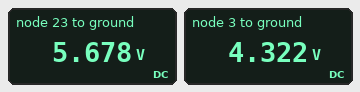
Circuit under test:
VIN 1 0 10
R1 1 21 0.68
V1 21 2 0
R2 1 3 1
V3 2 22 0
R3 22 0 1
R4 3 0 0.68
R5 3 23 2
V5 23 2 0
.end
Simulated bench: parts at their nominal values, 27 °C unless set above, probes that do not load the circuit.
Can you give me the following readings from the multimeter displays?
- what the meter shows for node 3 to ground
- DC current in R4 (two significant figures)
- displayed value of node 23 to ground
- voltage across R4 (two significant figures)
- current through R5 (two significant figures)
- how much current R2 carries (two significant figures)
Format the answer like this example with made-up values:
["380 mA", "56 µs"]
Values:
["4.322 V", "6.4 A", "5.678 V", "4.3 V", "680 mA", "5.7 A"]
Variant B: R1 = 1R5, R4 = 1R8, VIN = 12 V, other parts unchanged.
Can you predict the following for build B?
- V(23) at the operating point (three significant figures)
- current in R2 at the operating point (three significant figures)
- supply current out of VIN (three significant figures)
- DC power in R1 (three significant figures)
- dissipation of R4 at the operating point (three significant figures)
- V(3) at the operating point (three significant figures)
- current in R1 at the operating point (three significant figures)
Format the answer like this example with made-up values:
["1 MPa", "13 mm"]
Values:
["5.34 V", "4.86 A", "9.30 A", "29.6 W", "28.3 W", "7.14 V", "4.44 A"]
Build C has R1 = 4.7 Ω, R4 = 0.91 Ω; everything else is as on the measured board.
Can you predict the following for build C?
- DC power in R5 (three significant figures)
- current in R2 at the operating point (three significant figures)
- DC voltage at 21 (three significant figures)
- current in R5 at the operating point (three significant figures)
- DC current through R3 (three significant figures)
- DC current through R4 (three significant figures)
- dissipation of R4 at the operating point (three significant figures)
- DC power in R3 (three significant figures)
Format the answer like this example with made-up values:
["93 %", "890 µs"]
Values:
["1.66 W", "5.67 A", "2.51 V", "912 mA", "2.51 A", "4.76 A", "20.6 W", "6.28 W"]
